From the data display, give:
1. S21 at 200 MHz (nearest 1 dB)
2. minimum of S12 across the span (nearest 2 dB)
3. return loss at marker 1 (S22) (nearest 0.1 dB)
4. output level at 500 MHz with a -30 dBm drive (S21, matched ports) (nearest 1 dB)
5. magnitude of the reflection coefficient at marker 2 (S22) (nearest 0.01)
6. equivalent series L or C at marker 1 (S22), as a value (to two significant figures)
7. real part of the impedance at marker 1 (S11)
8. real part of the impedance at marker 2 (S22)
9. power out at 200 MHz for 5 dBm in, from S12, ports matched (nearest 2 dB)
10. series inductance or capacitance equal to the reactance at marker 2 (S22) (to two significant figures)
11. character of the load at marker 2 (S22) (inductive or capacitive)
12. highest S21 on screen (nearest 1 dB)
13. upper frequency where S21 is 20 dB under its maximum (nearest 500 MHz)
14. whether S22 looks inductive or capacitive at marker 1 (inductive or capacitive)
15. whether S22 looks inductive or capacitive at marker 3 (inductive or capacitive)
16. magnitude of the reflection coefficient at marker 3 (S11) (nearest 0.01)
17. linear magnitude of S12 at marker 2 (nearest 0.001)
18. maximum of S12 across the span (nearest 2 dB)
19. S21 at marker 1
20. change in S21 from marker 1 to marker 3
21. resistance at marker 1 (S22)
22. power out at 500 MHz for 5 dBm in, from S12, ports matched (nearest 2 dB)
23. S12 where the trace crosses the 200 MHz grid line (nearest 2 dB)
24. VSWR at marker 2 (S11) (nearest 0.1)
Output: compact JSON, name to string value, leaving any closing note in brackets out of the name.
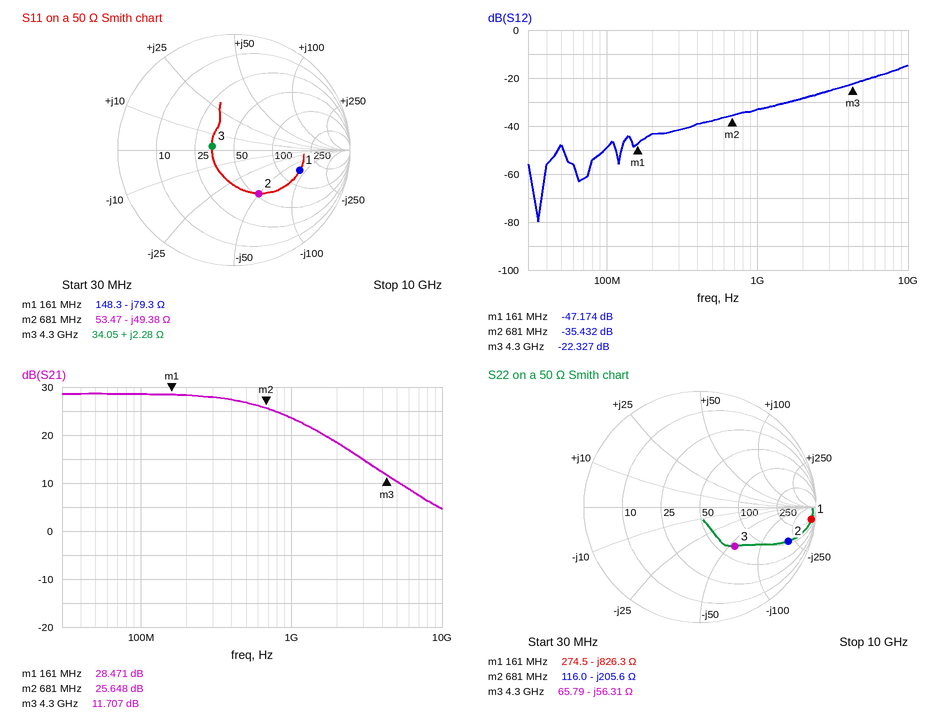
{"S21 at 200 MHz": "28 dB", "minimum of S12 across the span": "-80 dB", "return loss at marker 1 (S22)": "0.3 dB", "output level at 500 MHz with a -30 dBm drive (S21, matched ports)": "-3 dBm", "magnitude of the reflection coefficient at marker 2 (S22)": "0.82", "equivalent series L or C at marker 1 (S22), as a value": "1.2 pF", "real part of the impedance at marker 1": "148.3 Ω", "real part of the impedance at marker 2": "116.0 Ω", "power out at 200 MHz for 5 dBm in, from S12, ports matched": "-38 dBm", "series inductance or capacitance equal to the reactance at marker 2 (S22)": "1.1 pF", "character of the load at marker 2 (S22)": "capacitive", "highest S21 on screen": "29 dB", "upper frequency where S21 is 20 dB under its maximum": "6.0 GHz", "whether S22 looks inductive or capacitive at marker 1": "capacitive", "whether S22 looks inductive or capacitive at marker 3": "capacitive", "magnitude of the reflection coefficient at marker 3 (S11)": "0.19", "linear magnitude of S12 at marker 2": "0.017", "maximum of S12 across the span": "-14 dB", "S21 at marker 1": "28.471 dB", "change in S21 from marker 1 to marker 3": "-16.764 dB", "resistance at marker 1": "274.5 Ω", "power out at 500 MHz for 5 dBm in, from S12, ports matched": "-32 dBm", "S12 where the trace crosses the 200 MHz grid line": "-44 dB", "VSWR at marker 2 (S11)": "2.5"}
